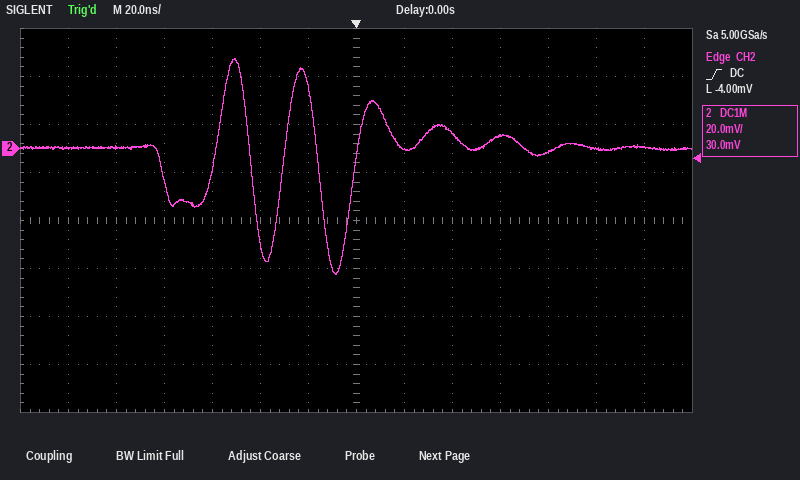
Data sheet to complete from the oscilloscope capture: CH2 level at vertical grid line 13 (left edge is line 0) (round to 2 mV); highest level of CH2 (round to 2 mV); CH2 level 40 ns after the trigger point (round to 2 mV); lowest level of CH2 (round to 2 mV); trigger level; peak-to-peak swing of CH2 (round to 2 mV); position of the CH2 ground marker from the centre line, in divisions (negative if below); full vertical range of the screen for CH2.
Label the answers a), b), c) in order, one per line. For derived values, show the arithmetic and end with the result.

a) 0 mV
b) 38 mV
c) 6 mV
d) -52 mV
e) -4.00 mV
f) 38 mV − (-52 mV) = 90 mV
g) +1.5 div
h) 160 mV
